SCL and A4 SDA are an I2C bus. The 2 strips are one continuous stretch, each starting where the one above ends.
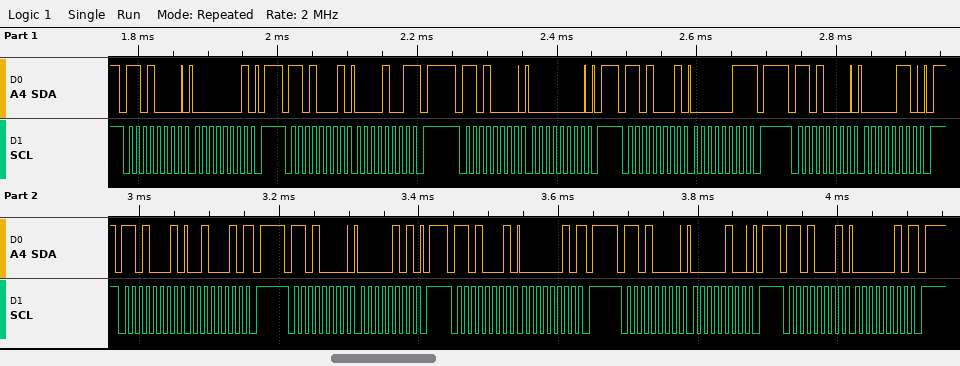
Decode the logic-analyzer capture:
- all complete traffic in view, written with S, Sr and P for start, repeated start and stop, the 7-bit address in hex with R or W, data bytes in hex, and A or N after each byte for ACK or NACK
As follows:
S 68W A 01 A P S 68R A 09 N P S 68W A 00 A P S 68R A 03 N P S 68W A 06 A P S 68R A 22 N P S 68W A 05 A P S 68R A 02 N P S 68W A 04 A P S 68R A 02 N P
